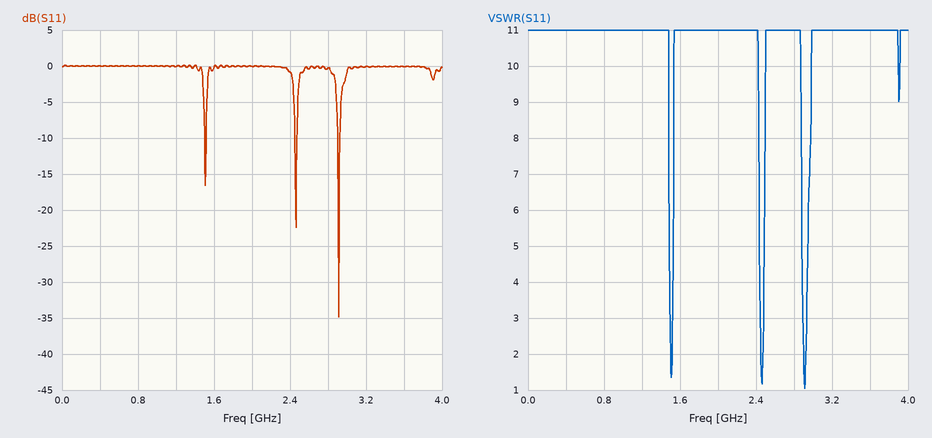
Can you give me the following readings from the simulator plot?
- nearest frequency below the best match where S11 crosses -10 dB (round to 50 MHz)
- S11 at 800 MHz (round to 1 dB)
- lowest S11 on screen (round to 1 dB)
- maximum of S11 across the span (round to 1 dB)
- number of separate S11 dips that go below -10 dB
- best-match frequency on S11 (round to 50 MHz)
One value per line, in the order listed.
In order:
2.90 GHz
0 dB
-35 dB
0 dB
3
2.90 GHz
